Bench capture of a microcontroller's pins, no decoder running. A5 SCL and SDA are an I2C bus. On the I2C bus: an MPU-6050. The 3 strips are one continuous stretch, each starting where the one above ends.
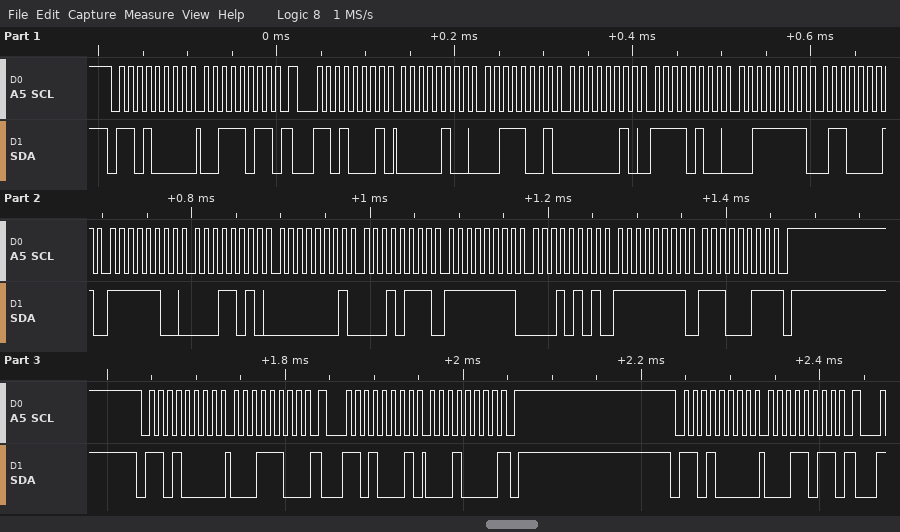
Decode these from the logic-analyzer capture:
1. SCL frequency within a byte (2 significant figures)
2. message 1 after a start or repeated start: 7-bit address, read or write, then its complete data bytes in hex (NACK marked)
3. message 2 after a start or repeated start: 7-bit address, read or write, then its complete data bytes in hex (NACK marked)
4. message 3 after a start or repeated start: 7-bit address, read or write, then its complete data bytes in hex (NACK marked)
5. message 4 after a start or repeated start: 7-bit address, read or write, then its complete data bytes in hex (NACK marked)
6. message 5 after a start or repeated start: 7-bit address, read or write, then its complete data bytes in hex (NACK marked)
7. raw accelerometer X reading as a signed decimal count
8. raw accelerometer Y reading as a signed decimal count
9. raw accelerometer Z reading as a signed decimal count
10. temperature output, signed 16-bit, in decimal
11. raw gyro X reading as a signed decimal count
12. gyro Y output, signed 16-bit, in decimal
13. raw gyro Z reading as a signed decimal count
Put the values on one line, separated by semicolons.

100 kHz; 0x68 write: 3B; 0x68 read: 04 39 02 F4 3F 61 FC 1A 01 17 FF 15 FF E3 NACK; 0x68 write: 1C; 0x68 read: 10 NACK; 0x68 write: 1B; 1081; 756; 16225; -998; 279; -235; -29
